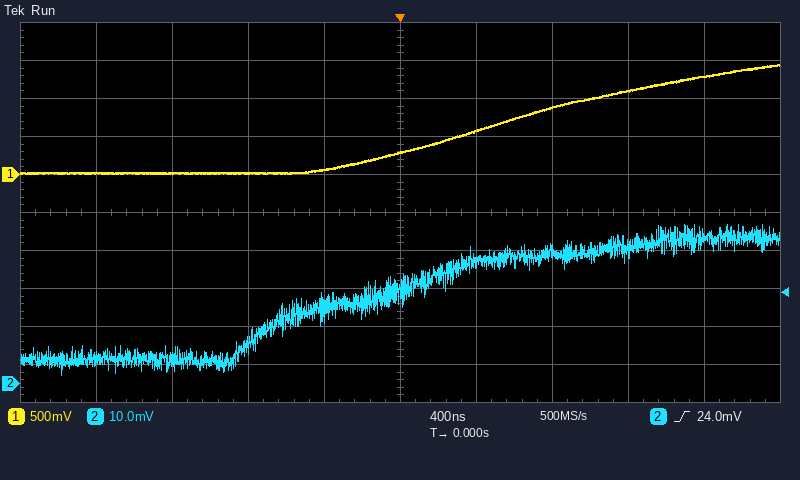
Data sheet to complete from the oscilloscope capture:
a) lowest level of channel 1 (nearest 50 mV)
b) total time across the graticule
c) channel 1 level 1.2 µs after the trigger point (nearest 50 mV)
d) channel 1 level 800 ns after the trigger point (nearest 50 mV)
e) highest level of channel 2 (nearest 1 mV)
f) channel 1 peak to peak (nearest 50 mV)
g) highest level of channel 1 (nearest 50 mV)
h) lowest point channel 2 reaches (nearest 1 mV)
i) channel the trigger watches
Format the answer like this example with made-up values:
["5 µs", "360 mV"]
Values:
["0 mV", "4 µs", "1.10 V", "900 mV", "42 mV", "1.45 V", "1.45 V", "2 mV", "channel 2"]
